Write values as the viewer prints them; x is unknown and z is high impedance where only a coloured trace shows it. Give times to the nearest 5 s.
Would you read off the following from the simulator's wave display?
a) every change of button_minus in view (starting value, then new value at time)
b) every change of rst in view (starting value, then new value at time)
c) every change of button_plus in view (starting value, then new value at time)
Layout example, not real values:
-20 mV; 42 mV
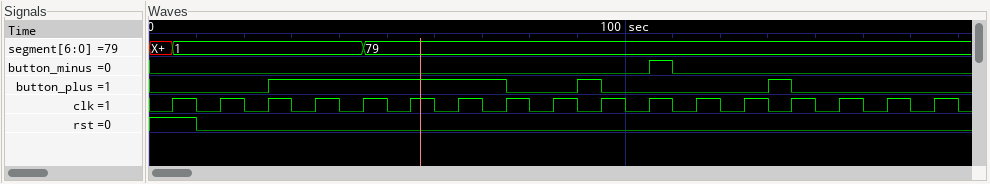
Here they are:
0, 1 at 105 s, 0 at 110 s; 1, 0 at 10 s; 0, 1 at 25 s, 0 at 75 s, 1 at 90 s, 0 at 95 s, 1 at 130 s, 0 at 135 s
